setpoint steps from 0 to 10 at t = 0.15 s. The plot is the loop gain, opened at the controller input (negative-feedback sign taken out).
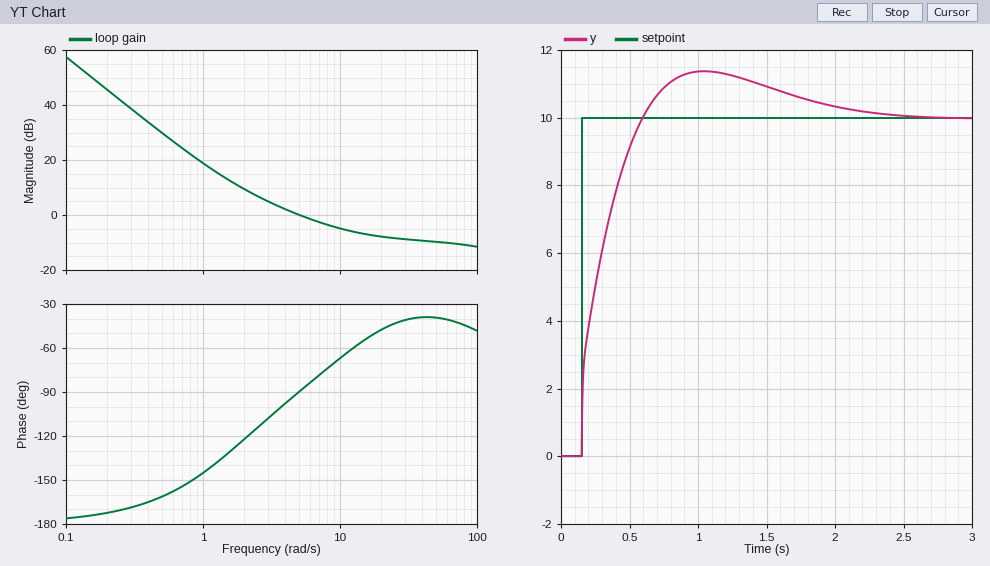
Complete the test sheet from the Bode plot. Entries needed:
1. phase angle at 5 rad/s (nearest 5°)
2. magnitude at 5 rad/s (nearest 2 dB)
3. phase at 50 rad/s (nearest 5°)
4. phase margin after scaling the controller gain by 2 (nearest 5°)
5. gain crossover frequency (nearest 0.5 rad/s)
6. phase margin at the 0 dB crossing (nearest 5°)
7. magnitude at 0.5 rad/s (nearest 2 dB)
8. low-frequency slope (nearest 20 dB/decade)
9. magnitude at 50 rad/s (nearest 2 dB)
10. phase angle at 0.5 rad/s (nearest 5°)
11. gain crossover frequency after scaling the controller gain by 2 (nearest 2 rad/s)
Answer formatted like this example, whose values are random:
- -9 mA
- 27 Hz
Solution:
- -90°
- 0 dB
- -40°
- 120°
- 5.0 rad/s
- 90°
- 30 dB
- -40 dB/decade
- -10 dB
- -160°
- 12 rad/s
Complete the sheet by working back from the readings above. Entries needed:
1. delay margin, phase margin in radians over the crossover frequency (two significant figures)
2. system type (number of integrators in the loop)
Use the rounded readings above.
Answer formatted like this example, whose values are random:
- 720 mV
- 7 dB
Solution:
- 0.31 s
- 2
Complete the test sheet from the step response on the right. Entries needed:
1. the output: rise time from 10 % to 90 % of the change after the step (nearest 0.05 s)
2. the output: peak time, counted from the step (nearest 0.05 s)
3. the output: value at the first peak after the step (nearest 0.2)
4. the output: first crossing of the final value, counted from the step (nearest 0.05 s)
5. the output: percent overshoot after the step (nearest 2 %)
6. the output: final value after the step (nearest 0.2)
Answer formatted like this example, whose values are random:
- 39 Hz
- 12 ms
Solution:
- 0.35 s
- 0.90 s
- 11.4
- 0.45 s
- 14 %
- 10.0
